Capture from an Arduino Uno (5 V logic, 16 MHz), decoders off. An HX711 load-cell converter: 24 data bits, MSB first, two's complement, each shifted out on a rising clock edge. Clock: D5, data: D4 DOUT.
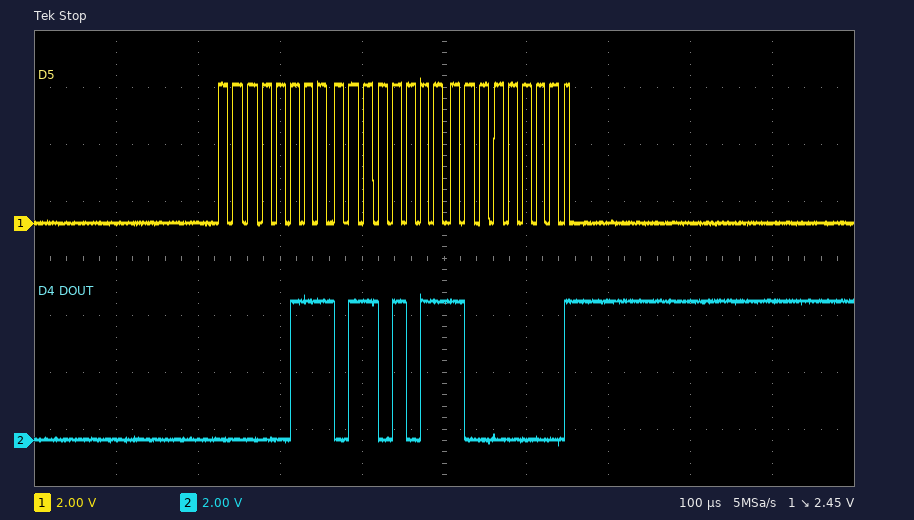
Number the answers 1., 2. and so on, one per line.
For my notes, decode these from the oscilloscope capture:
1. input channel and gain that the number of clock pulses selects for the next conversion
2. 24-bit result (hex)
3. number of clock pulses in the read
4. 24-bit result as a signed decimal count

1. channel A, gain 128
2. 0x076B80
3. 25
4. 486272
